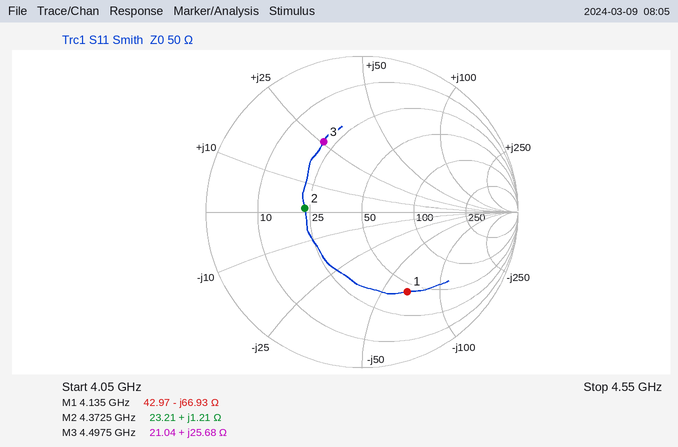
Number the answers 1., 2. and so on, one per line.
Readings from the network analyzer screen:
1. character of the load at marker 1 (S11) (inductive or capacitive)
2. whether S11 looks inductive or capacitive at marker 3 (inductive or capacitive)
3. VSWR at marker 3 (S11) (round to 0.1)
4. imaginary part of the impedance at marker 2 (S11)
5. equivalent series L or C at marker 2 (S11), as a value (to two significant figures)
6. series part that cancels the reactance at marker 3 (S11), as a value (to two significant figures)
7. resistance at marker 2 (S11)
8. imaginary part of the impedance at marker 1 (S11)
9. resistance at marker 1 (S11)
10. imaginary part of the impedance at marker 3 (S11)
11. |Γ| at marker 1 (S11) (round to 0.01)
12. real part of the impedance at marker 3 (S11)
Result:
1. capacitive
2. inductive
3. 3.1
4. +1.21 Ω
5. 44 pH
6. 1.4 pF
7. 23.21 Ω
8. -66.93 Ω
9. 42.97 Ω
10. +25.68 Ω
11. 0.59
12. 21.04 Ω
